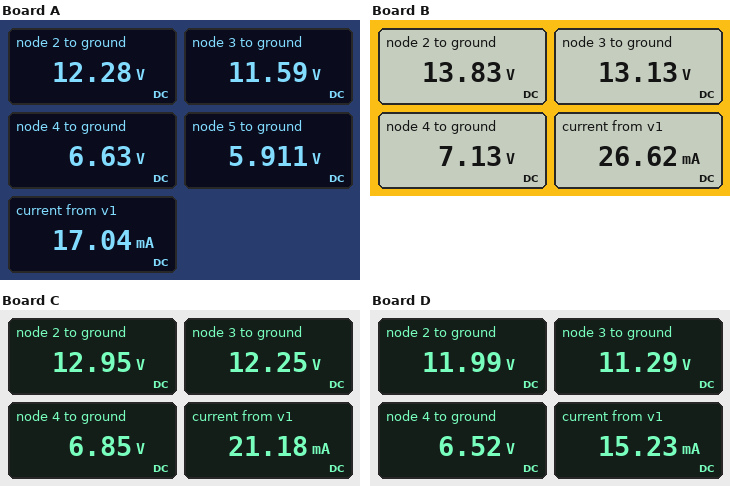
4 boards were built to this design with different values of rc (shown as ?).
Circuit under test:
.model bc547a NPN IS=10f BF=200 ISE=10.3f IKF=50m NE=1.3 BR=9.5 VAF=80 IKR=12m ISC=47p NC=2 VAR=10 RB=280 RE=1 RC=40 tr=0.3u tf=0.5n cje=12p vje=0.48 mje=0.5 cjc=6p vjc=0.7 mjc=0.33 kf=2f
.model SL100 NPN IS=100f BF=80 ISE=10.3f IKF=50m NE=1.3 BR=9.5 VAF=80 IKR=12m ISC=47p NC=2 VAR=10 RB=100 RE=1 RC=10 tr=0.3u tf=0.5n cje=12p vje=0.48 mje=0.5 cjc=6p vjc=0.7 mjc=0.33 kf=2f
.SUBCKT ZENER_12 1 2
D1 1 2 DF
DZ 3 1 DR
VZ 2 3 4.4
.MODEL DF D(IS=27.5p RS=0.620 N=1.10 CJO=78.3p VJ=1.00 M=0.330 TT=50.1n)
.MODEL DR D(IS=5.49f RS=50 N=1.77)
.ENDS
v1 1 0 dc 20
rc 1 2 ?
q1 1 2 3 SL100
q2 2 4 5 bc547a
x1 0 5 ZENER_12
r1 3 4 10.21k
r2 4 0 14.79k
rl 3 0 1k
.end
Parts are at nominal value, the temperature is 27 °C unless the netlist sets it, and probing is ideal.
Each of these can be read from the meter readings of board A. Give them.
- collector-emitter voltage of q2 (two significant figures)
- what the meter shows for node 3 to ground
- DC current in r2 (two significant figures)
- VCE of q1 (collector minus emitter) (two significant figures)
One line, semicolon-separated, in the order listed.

6.4 V; 11.59 V; 450 µA; 8.4 V
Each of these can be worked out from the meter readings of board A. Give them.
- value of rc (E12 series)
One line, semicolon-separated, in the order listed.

1.5 kΩ
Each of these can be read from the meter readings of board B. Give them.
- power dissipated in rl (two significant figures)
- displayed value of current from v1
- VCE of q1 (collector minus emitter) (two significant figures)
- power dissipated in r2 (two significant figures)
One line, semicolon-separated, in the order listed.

170 mW; 26.62 mA; 6.9 V; 3.4 mW
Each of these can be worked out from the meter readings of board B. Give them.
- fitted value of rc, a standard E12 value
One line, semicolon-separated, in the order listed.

470 Ω
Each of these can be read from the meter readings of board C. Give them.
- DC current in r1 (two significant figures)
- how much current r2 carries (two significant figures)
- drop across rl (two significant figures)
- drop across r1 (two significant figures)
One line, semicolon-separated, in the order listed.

530 µA; 460 µA; 12 V; 5.4 V
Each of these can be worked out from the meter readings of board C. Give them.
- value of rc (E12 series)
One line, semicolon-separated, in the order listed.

820 Ω
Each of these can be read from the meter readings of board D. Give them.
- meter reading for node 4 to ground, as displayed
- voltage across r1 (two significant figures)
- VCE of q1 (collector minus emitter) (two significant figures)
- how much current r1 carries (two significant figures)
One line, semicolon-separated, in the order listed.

6.52 V; 4.8 V; 8.7 V; 470 µA
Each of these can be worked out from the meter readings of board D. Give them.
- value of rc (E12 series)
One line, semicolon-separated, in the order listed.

2.2 kΩ
